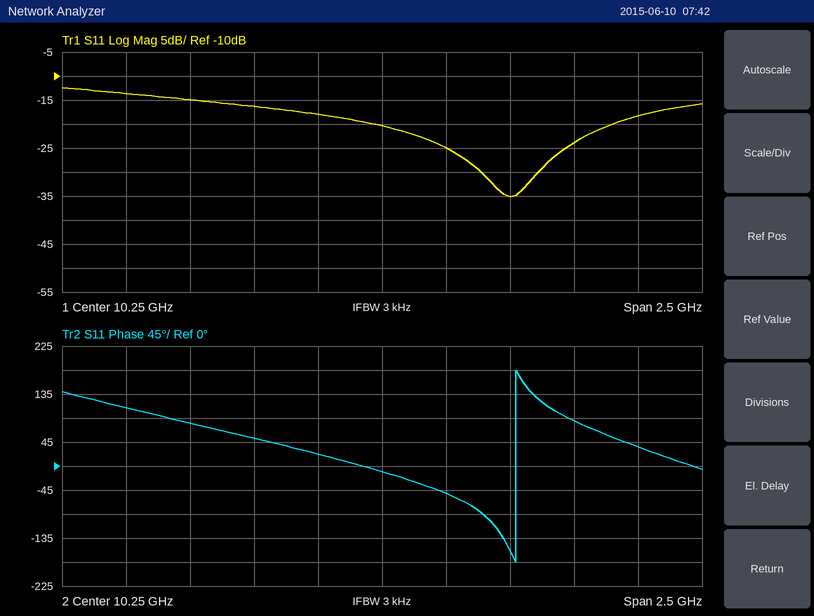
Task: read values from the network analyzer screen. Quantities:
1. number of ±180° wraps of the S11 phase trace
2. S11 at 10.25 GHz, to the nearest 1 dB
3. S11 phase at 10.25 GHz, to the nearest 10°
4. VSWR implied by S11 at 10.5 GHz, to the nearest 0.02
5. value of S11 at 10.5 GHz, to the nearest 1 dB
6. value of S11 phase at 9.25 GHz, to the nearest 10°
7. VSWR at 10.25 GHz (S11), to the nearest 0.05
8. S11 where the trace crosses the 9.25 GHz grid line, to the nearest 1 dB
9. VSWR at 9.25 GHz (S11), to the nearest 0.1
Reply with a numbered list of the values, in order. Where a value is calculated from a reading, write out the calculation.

1. 1
2. -20 dB
3. -10°
4. |Γ| = 10^(-25/20) = 0.0562; VSWR = (1 + 0.0562)/(1 − 0.0562) ≈ 1.12
5. -25 dB
6. 110°
7. |Γ| = 10^(-20/20) = 0.1000; VSWR = (1 + 0.1000)/(1 − 0.1000) ≈ 1.22, so 1.20 to the nearest 0.05
8. -14 dB
9. |Γ| = 10^(-14/20) = 0.1995; VSWR = (1 + 0.1995)/(1 − 0.1995) ≈ 1.5
